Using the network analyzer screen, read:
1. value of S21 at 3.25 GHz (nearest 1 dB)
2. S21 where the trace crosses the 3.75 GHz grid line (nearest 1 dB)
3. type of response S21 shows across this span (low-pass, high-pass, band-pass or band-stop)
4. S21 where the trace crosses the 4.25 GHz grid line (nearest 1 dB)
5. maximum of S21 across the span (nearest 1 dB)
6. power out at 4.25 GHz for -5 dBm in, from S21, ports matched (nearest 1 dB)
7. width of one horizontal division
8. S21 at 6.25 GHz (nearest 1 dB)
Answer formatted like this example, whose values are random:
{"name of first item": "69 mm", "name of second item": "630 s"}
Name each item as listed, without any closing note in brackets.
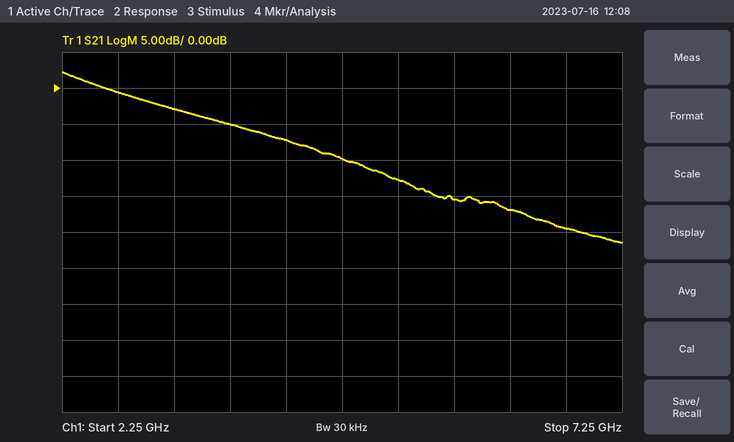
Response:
{"value of S21 at 3.25 GHz": "-3 dB", "S21 where the trace crosses the 3.75 GHz grid line": "-5 dB", "type of response S21 shows across this span": "low-pass", "S21 where the trace crosses the 4.25 GHz grid line": "-7 dB", "maximum of S21 across the span": "2 dB", "power out at 4.25 GHz for -5 dBm in, from S21, ports matched": "-12 dBm", "width of one horizontal division": "500 MHz", "S21 at 6.25 GHz": "-17 dB"}
